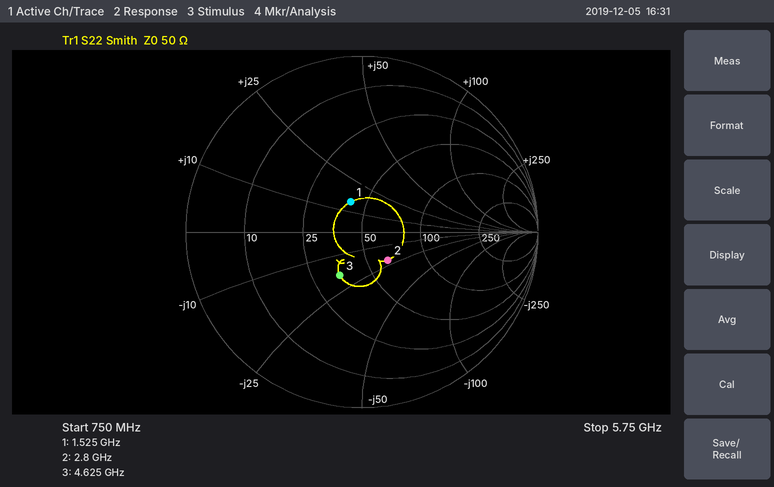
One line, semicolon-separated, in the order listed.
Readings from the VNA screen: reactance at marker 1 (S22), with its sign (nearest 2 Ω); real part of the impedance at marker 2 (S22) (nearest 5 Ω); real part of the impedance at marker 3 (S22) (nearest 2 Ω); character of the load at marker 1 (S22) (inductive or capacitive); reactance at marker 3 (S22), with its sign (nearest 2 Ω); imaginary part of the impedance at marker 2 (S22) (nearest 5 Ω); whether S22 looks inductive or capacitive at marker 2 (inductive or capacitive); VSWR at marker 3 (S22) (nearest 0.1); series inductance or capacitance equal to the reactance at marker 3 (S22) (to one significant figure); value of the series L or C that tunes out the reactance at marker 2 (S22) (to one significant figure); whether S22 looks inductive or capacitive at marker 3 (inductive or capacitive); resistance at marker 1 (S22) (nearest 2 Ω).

+14 Ω; 65 Ω; 34 Ω; inductive; -18 Ω; -20 Ω; capacitive; 1.8; 2 pF; 1 nH; capacitive; 42 Ω
